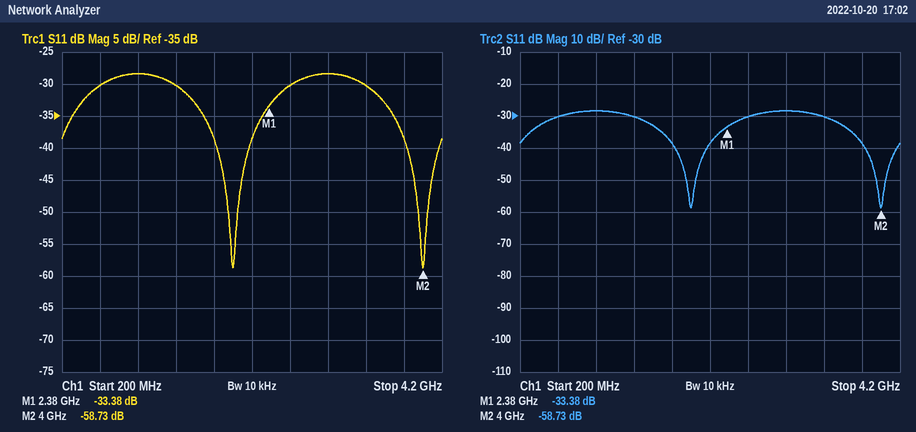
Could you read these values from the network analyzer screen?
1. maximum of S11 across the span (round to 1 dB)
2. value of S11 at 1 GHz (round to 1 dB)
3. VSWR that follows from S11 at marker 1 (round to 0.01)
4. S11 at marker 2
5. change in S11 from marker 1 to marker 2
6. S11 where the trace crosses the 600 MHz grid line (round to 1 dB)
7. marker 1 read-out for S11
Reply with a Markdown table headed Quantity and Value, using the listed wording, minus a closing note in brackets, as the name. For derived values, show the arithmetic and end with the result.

| Quantity | Value |
|---|---|
| maximum of S11 across the span | -28 dB |
| value of S11 at 1 GHz | -28 dB |
| VSWR that follows from S11 at marker 1 | (1 + 0.0214)/(1 − 0.0214) ≈ 1.04 |
| S11 at marker 2 | -58.73 dB |
| change in S11 from marker 1 to marker 2 | -58.73 − (-33.38) = -25.35 dB |
| S11 where the trace crosses the 600 MHz grid line | -30 dB |
| marker 1 read-out for S11 | -33.38 dB |
